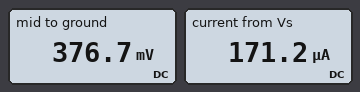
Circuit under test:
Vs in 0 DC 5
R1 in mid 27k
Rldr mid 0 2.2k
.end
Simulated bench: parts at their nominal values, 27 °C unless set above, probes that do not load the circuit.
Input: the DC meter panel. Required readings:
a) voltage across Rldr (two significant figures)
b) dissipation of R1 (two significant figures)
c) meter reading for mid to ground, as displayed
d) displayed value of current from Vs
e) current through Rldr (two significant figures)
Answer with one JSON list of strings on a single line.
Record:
["380 mV", "790 µW", "376.7 mV", "171.2 µA", "170 µA"]
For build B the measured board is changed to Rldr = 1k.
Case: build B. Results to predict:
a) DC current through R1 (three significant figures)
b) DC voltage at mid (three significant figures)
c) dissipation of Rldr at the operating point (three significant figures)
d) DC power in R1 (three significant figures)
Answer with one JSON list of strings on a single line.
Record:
["179 µA", "179 mV", "31.9 µW", "861 µW"]
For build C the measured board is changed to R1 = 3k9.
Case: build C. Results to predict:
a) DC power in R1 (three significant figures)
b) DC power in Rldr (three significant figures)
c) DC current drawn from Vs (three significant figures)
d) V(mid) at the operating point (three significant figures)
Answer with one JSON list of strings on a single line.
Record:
["2.62 mW", "1.48 mW", "820 µA", "1.80 V"]
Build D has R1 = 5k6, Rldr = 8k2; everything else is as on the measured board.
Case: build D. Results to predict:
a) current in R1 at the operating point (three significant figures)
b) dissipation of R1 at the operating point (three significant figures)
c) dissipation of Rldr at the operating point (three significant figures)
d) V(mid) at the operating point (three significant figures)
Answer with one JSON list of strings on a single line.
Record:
["362 µA", "735 µW", "1.08 mW", "2.97 V"]
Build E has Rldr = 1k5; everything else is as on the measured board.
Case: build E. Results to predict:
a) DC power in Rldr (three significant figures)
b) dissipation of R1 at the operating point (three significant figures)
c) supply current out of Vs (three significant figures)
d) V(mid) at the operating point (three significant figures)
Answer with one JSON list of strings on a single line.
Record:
["46.2 µW", "831 µW", "175 µA", "263 mV"]
